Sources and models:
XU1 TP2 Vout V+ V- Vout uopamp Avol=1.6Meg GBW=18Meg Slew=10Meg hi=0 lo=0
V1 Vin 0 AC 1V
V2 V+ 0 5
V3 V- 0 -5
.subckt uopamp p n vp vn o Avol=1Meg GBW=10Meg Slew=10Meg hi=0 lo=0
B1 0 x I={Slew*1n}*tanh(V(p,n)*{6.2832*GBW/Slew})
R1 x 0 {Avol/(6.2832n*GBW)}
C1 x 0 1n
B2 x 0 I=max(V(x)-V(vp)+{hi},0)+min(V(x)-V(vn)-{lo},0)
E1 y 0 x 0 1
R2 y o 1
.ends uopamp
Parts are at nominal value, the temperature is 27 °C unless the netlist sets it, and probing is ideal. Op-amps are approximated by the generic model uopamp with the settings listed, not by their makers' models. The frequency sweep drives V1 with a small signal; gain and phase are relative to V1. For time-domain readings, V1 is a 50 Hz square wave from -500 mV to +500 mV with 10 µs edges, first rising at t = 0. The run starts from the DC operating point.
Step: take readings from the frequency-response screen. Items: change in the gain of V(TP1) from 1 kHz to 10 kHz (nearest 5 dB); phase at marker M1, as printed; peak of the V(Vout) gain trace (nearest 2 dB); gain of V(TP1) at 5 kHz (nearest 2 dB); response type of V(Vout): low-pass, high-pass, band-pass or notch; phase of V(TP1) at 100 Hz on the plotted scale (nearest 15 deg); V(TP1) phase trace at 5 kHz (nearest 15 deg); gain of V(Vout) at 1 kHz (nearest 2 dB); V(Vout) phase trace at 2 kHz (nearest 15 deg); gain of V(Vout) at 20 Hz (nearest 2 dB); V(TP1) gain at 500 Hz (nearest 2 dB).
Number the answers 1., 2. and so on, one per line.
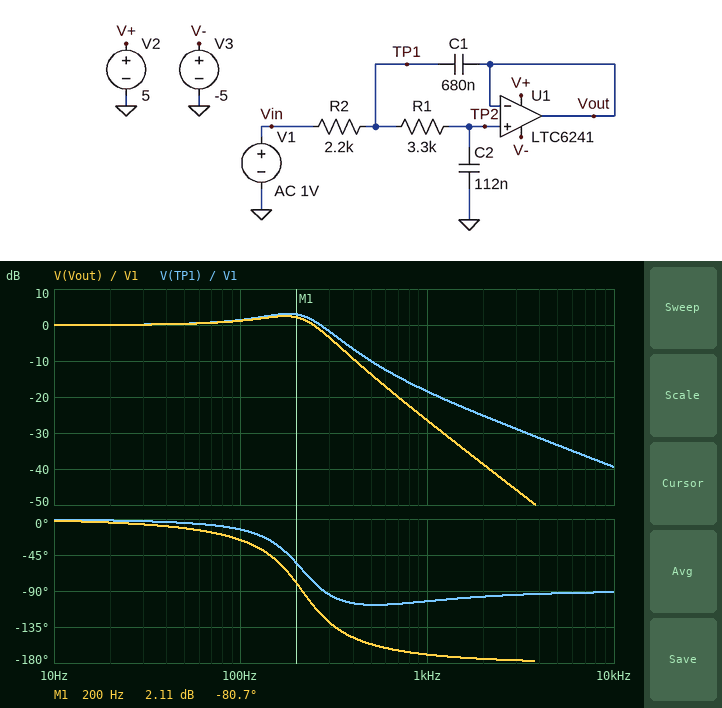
1. -20 dB
2. -80.7 deg
3. 2 dB
4. -34 dB
5. low-pass
6. -15 deg
7. -90 deg
8. -26 dB
9. -180 deg
10. 0 dB
11. -10 dB
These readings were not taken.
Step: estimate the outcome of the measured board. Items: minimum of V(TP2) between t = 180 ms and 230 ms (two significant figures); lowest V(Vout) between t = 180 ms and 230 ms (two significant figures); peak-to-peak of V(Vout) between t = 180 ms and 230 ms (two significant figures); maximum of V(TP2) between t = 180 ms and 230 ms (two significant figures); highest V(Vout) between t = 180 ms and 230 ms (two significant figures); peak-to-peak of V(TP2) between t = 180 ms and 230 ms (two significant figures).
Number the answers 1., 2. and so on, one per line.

1. -740 mV
2. -740 mV
3. 1.5 V
4. 740 mV
5. 740 mV
6. 1.5 V
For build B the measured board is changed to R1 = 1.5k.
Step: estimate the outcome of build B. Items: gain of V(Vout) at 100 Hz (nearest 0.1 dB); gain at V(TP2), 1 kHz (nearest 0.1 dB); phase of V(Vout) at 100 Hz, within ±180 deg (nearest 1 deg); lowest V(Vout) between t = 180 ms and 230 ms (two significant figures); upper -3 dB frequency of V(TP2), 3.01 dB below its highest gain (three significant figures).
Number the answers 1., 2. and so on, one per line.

1. 0.6 dB
2. -19.4 dB
3. -16 deg
4. -740 mV
5. 377 Hz
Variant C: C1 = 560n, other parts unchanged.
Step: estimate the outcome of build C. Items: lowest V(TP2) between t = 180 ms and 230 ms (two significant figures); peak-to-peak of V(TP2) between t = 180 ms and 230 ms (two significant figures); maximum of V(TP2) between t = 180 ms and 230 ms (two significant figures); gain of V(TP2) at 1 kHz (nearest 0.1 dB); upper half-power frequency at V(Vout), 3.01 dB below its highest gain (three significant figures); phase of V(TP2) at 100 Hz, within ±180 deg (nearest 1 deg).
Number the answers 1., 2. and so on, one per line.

1. -700 mV
2. 1.4 V
3. 700 mV
4. -24.8 dB
5. 279 Hz
6. -25 deg
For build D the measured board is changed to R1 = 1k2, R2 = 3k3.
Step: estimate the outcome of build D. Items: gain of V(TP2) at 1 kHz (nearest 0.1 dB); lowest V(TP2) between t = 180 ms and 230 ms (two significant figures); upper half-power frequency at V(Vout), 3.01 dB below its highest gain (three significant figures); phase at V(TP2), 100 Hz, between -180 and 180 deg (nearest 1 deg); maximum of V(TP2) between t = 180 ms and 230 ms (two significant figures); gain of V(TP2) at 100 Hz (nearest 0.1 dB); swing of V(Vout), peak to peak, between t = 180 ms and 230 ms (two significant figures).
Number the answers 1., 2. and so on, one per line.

1. -21.1 dB
2. -700 mV
3. 342 Hz
4. -20 deg
5. 700 mV
6. 0.6 dB
7. 1.4 V
